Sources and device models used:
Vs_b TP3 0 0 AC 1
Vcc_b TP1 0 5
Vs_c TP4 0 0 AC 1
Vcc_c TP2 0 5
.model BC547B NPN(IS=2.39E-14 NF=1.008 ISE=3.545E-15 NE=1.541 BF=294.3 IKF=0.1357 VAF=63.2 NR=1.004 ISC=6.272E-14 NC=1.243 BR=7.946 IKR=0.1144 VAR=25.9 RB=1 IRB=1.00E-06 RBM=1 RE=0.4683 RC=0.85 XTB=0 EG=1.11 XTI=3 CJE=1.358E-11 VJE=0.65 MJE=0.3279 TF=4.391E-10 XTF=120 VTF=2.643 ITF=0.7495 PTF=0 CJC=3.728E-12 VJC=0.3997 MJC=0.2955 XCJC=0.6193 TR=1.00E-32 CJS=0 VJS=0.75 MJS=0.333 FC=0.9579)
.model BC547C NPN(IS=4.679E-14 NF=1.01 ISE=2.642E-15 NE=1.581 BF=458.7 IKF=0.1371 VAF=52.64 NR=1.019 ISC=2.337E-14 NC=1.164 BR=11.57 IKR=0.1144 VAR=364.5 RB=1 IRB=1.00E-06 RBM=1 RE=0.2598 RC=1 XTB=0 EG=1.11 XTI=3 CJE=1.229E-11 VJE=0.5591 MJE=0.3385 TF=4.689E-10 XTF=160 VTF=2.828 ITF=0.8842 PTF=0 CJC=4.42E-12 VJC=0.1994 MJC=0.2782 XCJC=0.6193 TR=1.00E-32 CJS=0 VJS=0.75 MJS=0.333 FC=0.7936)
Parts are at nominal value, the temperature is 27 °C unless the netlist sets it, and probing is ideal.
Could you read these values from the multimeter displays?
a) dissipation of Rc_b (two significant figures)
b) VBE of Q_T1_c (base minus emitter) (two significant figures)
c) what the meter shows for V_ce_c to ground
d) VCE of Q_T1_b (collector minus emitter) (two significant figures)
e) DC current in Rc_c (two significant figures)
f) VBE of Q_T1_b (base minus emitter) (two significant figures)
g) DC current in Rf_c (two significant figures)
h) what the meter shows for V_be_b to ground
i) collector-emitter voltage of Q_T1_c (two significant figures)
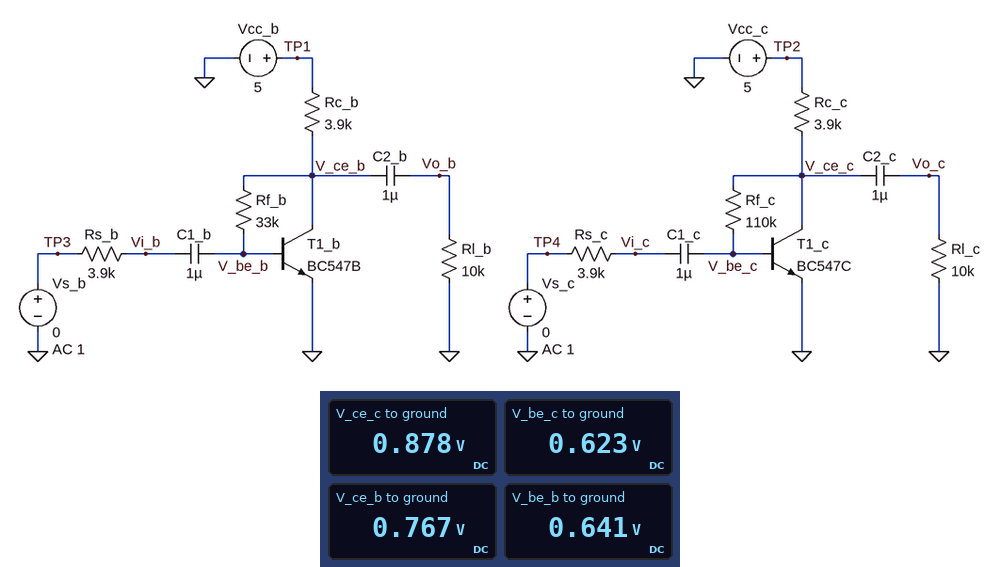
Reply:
4.6 mW
620 mV
0.878 V
770 mV
1.1 mA
640 mV
2.3 µA
0.641 V
880 mV
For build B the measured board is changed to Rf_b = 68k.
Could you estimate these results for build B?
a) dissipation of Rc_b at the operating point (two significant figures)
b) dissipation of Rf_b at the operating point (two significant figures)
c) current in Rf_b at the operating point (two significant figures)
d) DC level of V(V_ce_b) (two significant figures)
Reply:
4.3 mW
930 nW
3.7 µA
890 mV
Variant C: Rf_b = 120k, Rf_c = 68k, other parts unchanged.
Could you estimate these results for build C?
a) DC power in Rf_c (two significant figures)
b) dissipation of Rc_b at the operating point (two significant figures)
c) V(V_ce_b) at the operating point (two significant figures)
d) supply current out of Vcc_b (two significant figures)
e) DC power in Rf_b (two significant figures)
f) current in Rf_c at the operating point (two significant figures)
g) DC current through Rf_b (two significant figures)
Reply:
380 nW
4.0 mW
1.1 V
1.0 mA
1.5 µW
2.4 µA
3.5 µA
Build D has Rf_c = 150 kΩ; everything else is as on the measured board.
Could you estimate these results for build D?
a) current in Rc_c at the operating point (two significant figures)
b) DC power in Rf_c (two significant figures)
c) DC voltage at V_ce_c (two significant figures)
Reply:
1.0 mA
770 nW
960 mV
